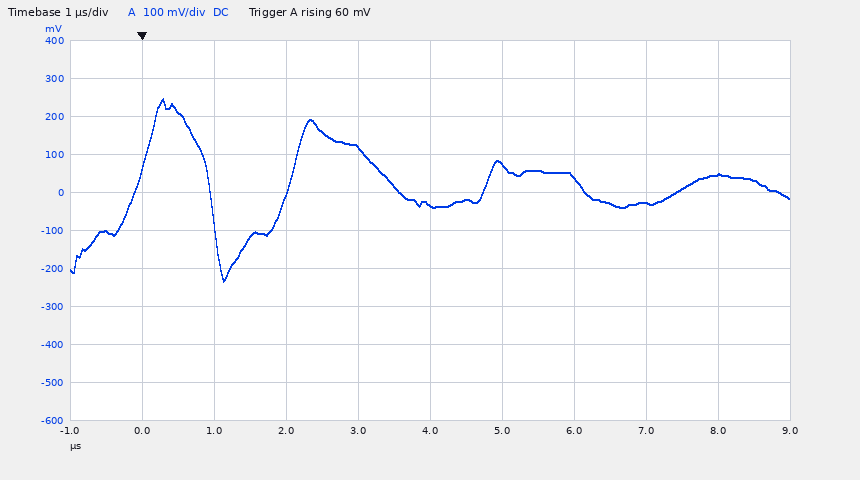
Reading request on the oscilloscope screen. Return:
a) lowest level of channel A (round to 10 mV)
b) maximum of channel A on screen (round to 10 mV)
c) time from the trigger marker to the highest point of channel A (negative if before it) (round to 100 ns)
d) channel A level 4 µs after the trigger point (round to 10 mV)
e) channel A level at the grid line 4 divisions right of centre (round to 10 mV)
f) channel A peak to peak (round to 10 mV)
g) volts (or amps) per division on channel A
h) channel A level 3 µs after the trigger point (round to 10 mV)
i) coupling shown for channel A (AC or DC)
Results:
-230 mV
250 mV
+300 ns
-30 mV
50 mV
480 mV
100 mV
120 mV
DC
